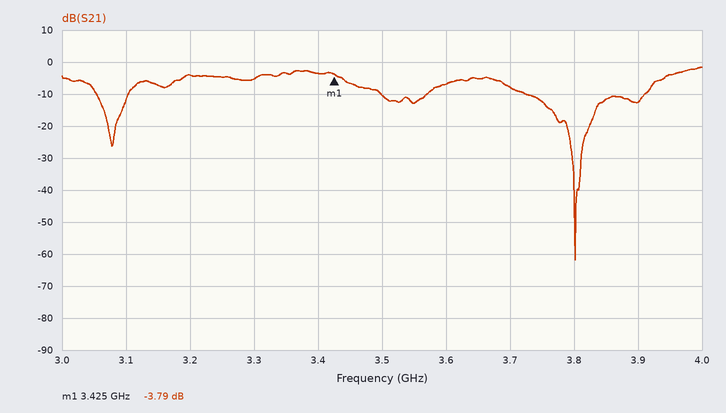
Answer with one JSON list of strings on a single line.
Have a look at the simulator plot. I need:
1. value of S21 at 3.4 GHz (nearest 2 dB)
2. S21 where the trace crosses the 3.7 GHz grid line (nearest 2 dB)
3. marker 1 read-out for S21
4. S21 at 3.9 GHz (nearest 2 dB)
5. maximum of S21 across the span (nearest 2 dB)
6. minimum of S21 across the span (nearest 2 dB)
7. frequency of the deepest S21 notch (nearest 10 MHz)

["-4 dB", "-8 dB", "-3.79 dB", "-12 dB", "-2 dB", "-62 dB", "3.80 GHz"]
